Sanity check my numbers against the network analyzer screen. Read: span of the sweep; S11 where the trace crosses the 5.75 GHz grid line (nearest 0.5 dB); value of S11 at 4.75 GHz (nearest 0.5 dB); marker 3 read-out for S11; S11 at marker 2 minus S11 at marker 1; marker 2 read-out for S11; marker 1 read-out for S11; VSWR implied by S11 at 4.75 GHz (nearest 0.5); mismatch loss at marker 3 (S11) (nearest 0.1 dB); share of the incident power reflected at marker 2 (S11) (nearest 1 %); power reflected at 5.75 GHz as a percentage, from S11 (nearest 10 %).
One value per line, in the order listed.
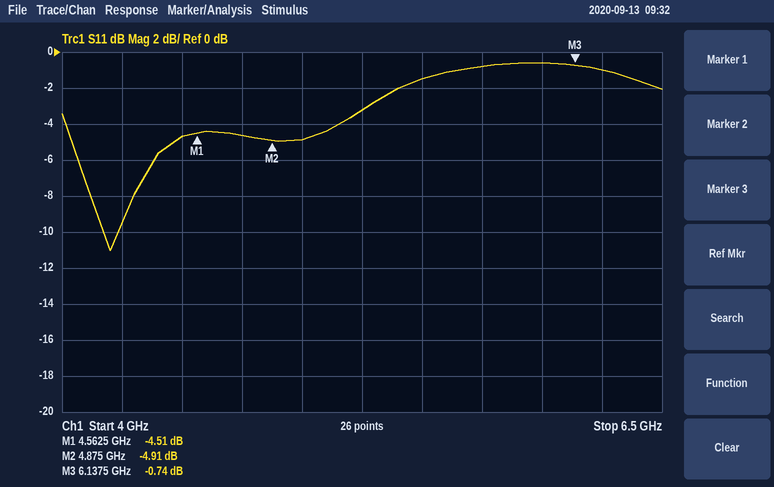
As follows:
2.5 GHz
-1.0 dB
-4.5 dB
-0.74 dB
-0.40 dB
-4.91 dB
-4.51 dB
4.0
8.1 dB
32 %
80 %
